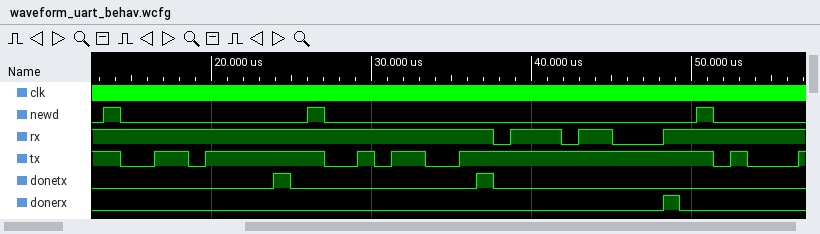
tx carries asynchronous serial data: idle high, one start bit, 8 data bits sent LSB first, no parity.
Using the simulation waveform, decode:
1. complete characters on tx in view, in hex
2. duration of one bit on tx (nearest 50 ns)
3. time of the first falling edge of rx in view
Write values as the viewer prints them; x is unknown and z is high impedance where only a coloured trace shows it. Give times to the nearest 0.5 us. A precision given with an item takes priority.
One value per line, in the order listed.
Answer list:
F6, 9A
1050 ns
37.5 us
